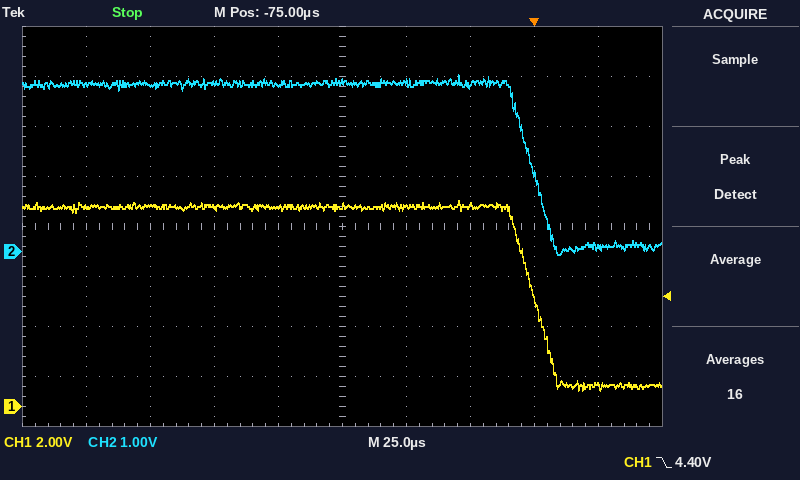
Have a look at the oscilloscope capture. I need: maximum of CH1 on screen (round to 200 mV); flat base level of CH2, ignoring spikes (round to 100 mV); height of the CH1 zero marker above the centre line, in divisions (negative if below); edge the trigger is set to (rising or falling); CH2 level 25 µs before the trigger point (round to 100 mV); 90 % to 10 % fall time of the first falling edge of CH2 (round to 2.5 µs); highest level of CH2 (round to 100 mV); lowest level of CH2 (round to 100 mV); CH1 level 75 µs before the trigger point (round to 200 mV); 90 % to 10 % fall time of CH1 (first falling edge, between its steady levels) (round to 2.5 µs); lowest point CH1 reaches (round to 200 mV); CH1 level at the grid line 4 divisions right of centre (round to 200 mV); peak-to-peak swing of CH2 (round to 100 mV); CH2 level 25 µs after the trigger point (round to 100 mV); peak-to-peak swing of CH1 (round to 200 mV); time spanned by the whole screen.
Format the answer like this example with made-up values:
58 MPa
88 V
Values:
8.2 V
100 mV
-3.6 div
falling
3.3 V
15.0 µs
3.5 V
-100 mV
8.0 V
15.0 µs
600 mV
800 mV
3.6 V
100 mV
7.6 V
250 µs
